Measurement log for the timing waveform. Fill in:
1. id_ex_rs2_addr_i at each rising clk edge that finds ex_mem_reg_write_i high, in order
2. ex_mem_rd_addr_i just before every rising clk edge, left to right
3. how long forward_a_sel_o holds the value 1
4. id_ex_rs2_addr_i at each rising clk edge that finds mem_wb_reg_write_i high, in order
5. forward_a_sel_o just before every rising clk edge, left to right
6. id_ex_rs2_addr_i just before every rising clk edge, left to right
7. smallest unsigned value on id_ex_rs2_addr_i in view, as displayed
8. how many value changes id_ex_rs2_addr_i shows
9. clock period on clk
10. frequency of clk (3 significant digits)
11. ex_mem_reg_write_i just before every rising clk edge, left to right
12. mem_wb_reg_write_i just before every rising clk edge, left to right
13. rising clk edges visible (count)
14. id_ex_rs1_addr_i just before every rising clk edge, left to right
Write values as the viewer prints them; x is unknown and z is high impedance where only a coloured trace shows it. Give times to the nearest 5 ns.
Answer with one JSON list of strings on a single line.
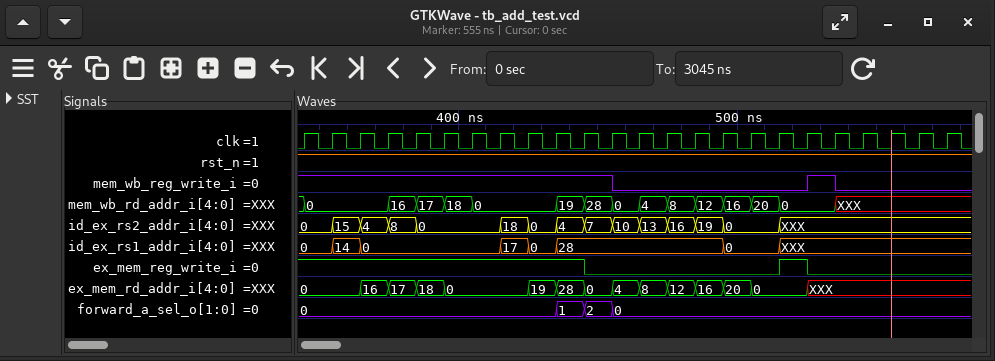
["0, 0, 15, 4, 8, 0, 0, 0, 18, 0, 4, XXX", "0, 0, 0, 16, 17, 18, 0, 0, 0, 19, 28, 0, 4, 8, 12, 16, 20, 0, 0, XXX, XXX, XXX, XXX, XXX", "10 ns", "0, 0, 15, 4, 8, 0, 0, 0, 18, 0, 4, 7, XXX", "0, 0, 0, 0, 0, 0, 0, 0, 0, 0, 1, 2, 0, 0, 0, 0, 0, 0, 0, 0, 0, 0, 0, 0", "0, 0, 15, 4, 8, 0, 0, 0, 18, 0, 4, 7, 10, 13, 16, 19, 0, 0, XXX, XXX, XXX, XXX, XXX, XXX", "0", "14", "10 ns", "100 MHz", "1 1 1 1 1 1 1 1 1 1 1 0 0 0 0 0 0 0 1 0 0 0 0 0", "1 1 1 1 1 1 1 1 1 1 1 1 0 0 0 0 0 0 0 1 0 0 0 0", "24", "0, 0, 14, 0, 0, 0, 0, 0, 17, 0, 28, 28, 28, 28, 28, 28, 0, 0, XXX, XXX, XXX, XXX, XXX, XXX"]
